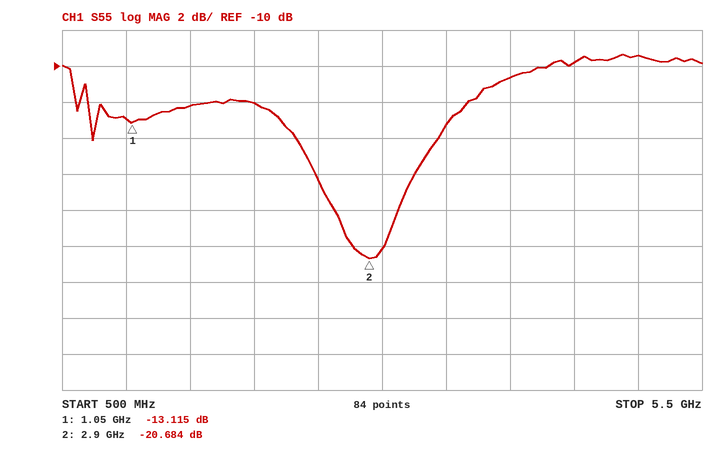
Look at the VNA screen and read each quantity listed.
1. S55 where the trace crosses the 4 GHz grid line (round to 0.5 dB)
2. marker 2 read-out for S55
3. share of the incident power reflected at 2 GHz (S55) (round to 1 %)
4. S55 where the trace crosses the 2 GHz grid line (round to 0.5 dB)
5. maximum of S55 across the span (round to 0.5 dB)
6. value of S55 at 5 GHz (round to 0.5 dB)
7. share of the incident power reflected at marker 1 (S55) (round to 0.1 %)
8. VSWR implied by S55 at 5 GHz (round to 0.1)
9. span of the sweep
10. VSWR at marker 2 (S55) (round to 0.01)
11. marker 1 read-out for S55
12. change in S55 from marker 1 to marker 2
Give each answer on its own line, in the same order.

-10.5 dB
-20.684 dB
6 %
-12.0 dB
-9.5 dB
-9.5 dB
4.9 %
2.0
5 GHz
1.20
-13.115 dB
-7.569 dB
